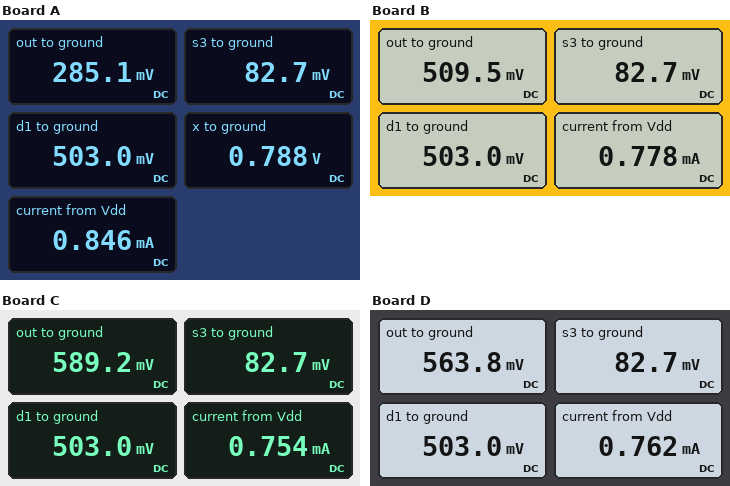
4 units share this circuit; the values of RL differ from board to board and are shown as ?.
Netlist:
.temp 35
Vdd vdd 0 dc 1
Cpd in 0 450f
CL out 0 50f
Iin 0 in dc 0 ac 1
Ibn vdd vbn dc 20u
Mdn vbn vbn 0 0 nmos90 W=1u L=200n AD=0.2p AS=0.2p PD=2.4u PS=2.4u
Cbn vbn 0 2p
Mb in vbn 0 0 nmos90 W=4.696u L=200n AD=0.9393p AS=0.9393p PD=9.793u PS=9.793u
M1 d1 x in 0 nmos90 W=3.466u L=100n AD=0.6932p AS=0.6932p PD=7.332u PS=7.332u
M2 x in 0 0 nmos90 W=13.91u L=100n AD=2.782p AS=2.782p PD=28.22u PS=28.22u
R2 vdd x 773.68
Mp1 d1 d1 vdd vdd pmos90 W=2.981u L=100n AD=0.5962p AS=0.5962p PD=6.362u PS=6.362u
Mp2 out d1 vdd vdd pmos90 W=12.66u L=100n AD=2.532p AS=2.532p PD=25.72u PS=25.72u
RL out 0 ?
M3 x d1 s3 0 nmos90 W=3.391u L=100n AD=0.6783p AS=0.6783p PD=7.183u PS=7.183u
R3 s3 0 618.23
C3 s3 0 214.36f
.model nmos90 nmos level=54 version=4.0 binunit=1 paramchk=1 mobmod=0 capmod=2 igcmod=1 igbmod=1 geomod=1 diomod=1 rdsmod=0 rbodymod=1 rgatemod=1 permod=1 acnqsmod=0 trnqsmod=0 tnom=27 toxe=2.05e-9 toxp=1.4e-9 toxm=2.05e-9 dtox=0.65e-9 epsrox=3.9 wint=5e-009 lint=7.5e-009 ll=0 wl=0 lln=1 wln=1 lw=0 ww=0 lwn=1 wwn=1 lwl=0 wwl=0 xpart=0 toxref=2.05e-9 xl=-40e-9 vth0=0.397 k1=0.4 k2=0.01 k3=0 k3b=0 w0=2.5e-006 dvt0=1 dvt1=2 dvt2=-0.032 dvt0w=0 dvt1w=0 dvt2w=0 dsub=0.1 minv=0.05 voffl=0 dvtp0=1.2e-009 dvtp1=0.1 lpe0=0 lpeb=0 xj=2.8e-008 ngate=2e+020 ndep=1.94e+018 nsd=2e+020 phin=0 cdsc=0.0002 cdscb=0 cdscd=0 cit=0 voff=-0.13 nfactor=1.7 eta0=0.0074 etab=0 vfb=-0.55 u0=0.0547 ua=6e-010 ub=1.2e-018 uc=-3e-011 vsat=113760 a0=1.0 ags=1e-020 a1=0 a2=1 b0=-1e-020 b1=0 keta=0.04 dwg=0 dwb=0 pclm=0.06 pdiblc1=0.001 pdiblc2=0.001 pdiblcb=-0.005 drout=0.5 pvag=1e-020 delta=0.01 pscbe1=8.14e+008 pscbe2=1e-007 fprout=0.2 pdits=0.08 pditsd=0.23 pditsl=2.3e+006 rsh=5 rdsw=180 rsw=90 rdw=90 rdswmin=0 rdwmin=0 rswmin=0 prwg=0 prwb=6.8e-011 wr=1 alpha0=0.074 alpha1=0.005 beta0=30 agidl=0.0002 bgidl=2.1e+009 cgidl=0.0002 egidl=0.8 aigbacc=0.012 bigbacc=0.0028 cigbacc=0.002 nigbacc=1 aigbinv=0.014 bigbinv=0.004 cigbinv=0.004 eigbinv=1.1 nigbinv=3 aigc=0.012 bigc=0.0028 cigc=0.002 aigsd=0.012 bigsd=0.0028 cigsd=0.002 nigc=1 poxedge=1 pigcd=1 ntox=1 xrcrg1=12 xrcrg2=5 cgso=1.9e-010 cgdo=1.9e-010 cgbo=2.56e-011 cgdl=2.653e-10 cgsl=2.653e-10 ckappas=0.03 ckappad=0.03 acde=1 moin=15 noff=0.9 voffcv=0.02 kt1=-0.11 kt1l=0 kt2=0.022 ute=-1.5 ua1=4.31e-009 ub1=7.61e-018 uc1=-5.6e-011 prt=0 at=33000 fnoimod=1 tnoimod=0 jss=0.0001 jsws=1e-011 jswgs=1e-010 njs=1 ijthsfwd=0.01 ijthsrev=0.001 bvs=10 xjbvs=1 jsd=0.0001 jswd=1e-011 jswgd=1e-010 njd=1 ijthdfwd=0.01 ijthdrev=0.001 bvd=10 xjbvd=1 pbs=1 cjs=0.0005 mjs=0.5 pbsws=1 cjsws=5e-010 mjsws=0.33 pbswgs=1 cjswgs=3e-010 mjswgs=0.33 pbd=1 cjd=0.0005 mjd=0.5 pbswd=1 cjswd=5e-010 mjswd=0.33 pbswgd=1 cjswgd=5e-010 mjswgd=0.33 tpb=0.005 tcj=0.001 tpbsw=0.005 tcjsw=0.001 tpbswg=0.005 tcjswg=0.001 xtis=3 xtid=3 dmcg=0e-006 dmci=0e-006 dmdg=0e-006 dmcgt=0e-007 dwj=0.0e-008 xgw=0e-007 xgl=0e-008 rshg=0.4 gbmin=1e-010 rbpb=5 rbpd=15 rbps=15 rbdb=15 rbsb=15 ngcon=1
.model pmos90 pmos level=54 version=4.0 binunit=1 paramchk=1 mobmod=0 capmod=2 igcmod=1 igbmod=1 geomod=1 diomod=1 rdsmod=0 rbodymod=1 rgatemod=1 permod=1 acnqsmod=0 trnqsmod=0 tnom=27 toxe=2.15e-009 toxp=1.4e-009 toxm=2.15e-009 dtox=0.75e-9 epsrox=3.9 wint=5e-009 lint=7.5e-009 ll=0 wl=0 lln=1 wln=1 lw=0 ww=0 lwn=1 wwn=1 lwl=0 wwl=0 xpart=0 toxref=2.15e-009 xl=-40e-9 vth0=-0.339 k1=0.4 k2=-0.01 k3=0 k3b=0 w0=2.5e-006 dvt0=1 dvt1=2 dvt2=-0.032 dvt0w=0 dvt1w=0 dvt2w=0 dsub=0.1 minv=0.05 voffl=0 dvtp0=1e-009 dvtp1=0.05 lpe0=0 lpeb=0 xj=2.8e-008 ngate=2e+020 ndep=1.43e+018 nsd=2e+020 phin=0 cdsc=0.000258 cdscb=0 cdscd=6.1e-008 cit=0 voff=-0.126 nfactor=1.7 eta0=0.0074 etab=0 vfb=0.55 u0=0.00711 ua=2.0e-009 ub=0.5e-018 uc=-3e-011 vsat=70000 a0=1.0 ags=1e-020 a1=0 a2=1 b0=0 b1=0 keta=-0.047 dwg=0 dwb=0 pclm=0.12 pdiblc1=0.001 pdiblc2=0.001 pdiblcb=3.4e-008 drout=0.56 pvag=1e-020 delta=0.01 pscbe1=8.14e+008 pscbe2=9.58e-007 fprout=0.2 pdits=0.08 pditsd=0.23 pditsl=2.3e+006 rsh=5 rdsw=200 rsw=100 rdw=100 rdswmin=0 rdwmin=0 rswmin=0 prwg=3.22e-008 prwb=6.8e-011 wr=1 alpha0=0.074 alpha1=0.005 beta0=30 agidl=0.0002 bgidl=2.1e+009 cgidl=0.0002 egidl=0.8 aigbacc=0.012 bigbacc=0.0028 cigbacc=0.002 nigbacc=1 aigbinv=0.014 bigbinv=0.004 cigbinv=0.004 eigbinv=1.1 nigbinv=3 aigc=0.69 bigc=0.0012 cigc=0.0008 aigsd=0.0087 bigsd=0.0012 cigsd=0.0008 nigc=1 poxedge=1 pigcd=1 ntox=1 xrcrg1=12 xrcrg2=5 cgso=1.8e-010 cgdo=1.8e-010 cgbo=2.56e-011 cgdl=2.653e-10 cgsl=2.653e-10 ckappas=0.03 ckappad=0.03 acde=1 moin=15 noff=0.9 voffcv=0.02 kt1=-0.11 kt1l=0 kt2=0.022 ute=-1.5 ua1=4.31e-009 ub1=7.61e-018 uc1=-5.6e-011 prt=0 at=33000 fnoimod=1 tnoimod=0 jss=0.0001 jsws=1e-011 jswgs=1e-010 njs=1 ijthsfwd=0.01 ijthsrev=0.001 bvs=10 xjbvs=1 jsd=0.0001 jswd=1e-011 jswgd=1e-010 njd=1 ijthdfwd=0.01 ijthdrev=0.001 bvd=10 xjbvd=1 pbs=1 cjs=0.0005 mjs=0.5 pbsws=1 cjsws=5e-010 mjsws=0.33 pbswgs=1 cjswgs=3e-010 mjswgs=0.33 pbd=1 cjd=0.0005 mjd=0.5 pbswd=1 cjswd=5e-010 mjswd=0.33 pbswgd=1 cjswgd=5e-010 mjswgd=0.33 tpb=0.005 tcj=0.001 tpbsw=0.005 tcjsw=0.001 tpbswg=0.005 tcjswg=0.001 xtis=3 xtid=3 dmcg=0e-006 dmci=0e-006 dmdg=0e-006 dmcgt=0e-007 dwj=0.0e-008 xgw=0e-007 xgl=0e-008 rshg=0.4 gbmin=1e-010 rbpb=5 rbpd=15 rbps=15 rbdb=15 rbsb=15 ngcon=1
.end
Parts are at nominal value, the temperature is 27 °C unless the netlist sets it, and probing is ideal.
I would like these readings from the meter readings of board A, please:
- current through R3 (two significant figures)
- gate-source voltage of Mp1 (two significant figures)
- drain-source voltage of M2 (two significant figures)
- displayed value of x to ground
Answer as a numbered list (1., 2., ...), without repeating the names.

1. 130 µA
2. -500 mV
3. 790 mV
4. 0.788 V
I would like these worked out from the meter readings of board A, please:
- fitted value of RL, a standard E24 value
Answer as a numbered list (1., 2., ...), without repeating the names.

1. 620 Ω
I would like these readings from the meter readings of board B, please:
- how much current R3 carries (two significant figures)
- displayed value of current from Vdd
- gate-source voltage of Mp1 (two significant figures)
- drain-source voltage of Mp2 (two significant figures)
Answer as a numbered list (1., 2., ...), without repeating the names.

1. 130 µA
2. 0.778 mA
3. -500 mV
4. -490 mV
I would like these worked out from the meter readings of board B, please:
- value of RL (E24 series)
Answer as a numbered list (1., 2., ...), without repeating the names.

1. 1.3 kΩ
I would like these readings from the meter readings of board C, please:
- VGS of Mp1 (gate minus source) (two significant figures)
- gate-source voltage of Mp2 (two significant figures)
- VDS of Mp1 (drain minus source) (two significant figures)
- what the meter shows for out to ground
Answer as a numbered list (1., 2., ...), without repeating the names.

1. -500 mV
2. -500 mV
3. -500 mV
4. 589.2 mV
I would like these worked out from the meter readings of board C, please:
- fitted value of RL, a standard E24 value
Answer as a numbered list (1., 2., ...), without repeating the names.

1. 1.6 kΩ
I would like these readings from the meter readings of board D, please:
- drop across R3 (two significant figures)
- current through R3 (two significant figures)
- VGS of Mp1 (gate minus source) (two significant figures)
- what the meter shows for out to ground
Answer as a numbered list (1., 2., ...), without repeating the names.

1. 83 mV
2. 130 µA
3. -500 mV
4. 563.8 mV
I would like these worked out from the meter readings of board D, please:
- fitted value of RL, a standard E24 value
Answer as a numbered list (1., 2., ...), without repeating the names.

1. 1.5 kΩ
